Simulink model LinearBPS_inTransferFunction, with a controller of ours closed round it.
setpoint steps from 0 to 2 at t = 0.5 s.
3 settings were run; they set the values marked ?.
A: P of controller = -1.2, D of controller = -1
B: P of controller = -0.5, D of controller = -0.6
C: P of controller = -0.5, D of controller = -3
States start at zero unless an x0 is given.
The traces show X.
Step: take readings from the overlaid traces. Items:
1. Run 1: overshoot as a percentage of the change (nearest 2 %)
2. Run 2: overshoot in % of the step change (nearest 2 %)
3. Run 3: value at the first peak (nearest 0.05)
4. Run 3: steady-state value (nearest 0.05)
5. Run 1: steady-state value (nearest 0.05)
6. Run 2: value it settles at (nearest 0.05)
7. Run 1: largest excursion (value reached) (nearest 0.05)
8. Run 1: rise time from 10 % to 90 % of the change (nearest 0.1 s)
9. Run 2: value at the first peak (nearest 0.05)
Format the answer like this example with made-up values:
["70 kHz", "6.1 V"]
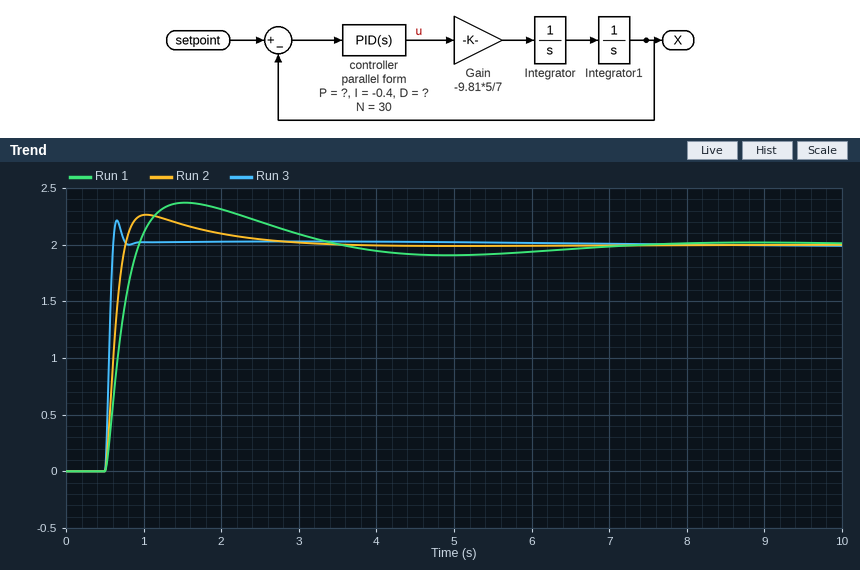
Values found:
["18 %", "14 %", "2.20", "2.00", "2.00", "2.00", "2.35", "0.3 s", "2.25"]
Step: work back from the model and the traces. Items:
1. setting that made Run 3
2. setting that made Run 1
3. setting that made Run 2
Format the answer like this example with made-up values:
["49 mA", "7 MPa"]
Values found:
["C", "B", "A"]
